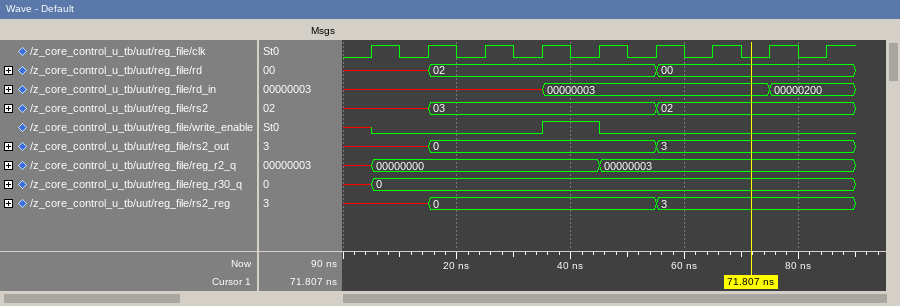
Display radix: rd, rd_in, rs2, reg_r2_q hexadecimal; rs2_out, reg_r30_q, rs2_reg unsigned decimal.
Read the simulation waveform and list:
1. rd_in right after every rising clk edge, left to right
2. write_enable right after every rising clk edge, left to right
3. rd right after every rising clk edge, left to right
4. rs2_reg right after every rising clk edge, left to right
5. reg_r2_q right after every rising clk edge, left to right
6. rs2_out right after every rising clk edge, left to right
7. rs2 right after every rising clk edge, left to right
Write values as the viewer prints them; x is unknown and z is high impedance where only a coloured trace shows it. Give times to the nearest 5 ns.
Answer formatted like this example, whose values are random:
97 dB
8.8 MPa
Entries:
x, x, x, 00000003, 00000003, 00000003, 00000003, 00000200, 00000200
0 0 0 1 0 0 0 0 0
x, 02, 02, 02, 02, 00, 00, 00, 00
x, 0, 0, 0, 0, 3, 3, 3, 3
00000000, 00000000, 00000000, 00000000, 00000003, 00000003, 00000003, 00000003, 00000003
x, 0, 0, 0, 0, 3, 3, 3, 3
x, 03, 03, 03, 03, 02, 02, 02, 02
